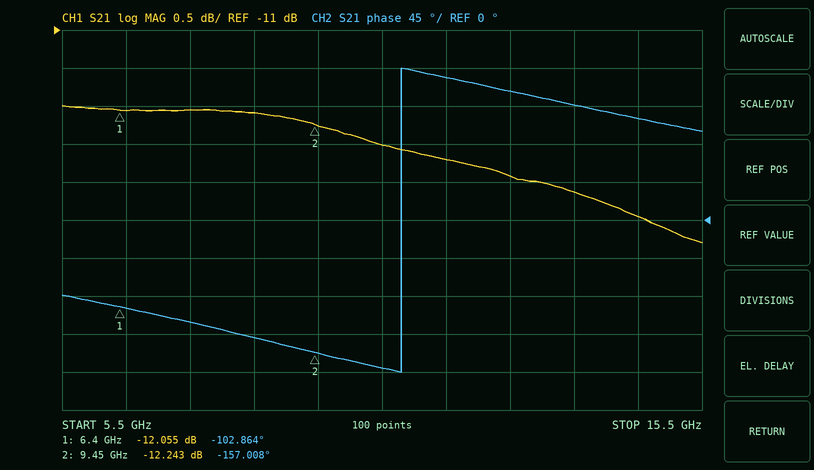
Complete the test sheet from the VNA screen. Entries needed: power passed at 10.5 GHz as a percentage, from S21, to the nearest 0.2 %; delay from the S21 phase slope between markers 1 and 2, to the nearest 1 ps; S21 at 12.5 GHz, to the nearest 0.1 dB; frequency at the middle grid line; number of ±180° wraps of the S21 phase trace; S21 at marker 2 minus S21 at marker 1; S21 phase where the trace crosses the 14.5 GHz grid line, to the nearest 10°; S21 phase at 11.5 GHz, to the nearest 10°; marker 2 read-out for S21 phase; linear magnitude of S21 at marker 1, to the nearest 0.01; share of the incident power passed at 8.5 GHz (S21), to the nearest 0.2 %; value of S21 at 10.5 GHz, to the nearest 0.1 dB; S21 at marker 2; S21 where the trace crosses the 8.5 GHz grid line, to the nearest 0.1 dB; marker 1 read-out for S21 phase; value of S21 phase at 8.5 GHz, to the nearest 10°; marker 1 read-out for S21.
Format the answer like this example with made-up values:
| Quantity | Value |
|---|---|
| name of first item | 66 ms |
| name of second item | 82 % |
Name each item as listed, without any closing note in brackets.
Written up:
| Quantity | Value |
|---|---|
| power passed at 10.5 GHz as a percentage, from S21, to the nearest 0.2 % | 5.6 % |
| delay from the S21 phase slope between markers 1 and 2, to the nearest 1 ps | 49 ps |
| S21 at 12.5 GHz, to the nearest 0.1 dB | -12.9 dB |
| frequency at the middle grid line | 10.5 GHz |
| number of ±180° wraps of the S21 phase trace | 1 |
| S21 at marker 2 minus S21 at marker 1 | -0.188 dB |
| S21 phase where the trace crosses the 14.5 GHz grid line, to the nearest 10° | 120° |
| S21 phase at 11.5 GHz, to the nearest 10° | 170° |
| marker 2 read-out for S21 phase | -157.008° |
| linear magnitude of S21 at marker 1, to the nearest 0.01 | 0.25 |
| share of the incident power passed at 8.5 GHz (S21), to the nearest 0.2 % | 6.2 % |
| value of S21 at 10.5 GHz, to the nearest 0.1 dB | -12.5 dB |
| S21 at marker 2 | -12.243 dB |
| S21 where the trace crosses the 8.5 GHz grid line, to the nearest 0.1 dB | -12.1 dB |
| marker 1 read-out for S21 phase | -102.864° |
| value of S21 phase at 8.5 GHz, to the nearest 10° | -140° |
| marker 1 read-out for S21 | -12.055 dB |
